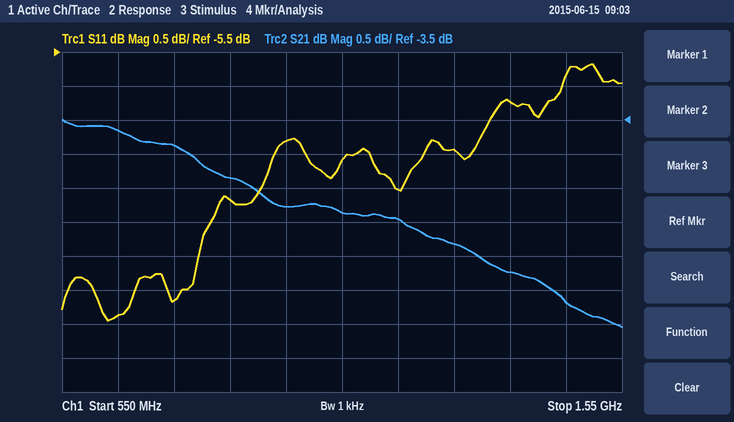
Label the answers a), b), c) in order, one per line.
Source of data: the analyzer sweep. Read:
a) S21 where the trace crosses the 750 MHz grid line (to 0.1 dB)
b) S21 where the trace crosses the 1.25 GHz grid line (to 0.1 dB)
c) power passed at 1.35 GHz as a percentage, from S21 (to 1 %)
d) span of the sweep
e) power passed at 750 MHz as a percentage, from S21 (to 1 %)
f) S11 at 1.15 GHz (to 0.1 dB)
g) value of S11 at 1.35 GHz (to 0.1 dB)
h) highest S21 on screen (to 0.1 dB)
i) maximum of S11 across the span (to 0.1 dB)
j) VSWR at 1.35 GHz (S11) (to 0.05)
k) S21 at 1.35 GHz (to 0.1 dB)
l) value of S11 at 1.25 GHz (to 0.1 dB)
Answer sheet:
a) -3.9 dB
b) -5.3 dB
c) 27 %
d) 1 GHz
e) 41 %
f) -7.5 dB
g) -6.2 dB
h) -3.5 dB
i) -5.7 dB
j) 2.90
k) -5.7 dB
l) -6.9 dB
